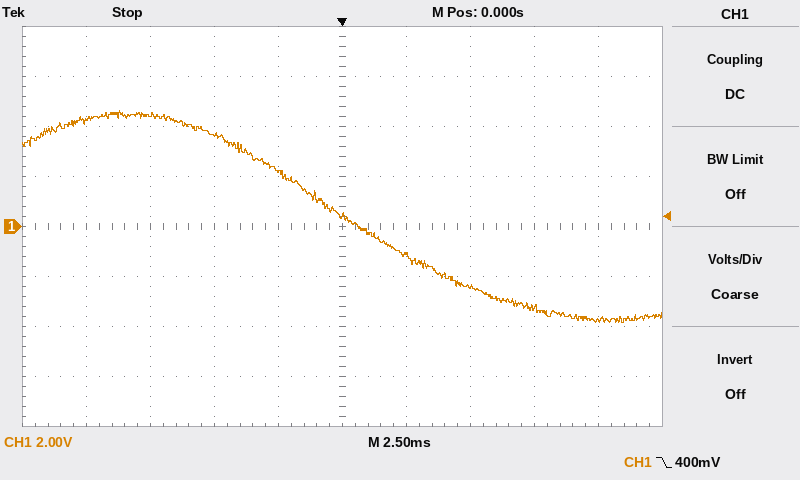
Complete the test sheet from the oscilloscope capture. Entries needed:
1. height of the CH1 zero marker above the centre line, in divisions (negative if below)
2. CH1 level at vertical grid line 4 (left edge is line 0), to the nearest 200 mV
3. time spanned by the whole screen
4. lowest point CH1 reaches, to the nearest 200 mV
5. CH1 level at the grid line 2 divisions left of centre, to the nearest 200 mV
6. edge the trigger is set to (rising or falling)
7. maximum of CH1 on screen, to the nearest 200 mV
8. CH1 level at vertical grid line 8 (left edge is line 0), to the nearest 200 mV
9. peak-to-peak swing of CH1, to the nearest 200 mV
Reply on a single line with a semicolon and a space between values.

0.0 div; 2.2 V; 25 ms; -3.8 V; 3.6 V; falling; 4.6 V; -3.2 V; 8.4 V
